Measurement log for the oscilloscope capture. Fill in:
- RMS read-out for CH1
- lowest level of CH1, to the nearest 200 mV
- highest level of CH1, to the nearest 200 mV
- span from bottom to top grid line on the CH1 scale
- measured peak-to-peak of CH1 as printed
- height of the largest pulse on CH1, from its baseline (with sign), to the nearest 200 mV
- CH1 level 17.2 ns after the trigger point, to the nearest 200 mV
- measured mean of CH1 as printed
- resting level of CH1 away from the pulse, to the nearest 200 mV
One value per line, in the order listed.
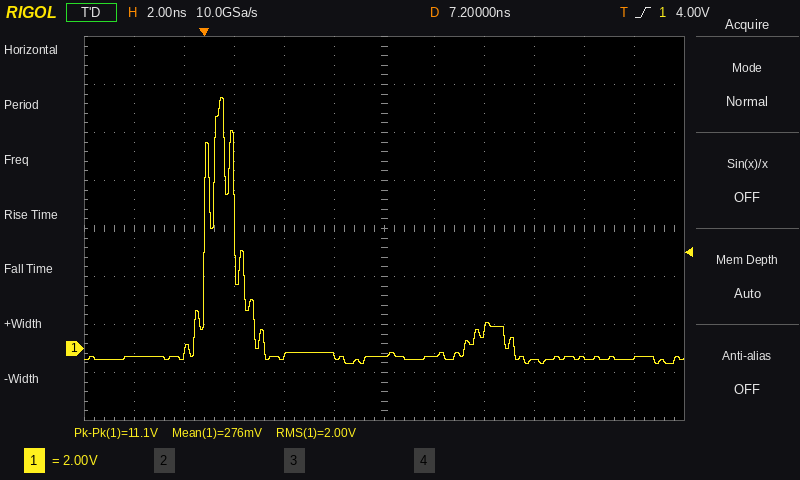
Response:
2.00 V
-600 mV
10.4 V
16 V
11.1 V
+10.8 V
-400 mV
276 mV
-400 mV
